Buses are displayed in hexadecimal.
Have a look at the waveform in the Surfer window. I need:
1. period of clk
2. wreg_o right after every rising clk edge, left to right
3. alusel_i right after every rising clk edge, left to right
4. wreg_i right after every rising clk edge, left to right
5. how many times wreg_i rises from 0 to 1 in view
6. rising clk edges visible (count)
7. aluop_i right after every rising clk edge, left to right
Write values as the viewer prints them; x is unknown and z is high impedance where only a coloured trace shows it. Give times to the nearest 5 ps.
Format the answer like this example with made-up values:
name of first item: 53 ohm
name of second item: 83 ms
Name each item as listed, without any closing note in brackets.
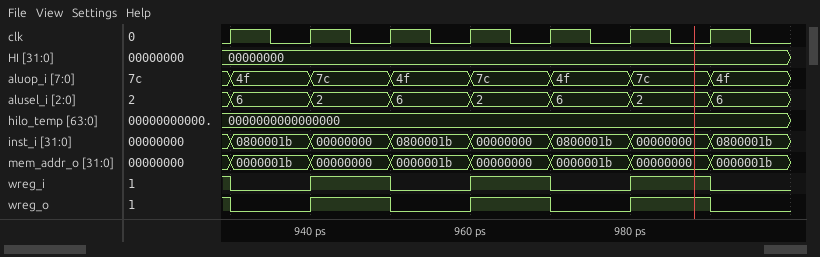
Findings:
period of clk: 10 ps
wreg_o right after every rising clk edge, left to right: 0 1 0 1 0 1 0
alusel_i right after every rising clk edge, left to right: 6, 2, 6, 2, 6, 2, 6
wreg_i right after every rising clk edge, left to right: 0 1 0 1 0 1 0
how many times wreg_i rises from 0 to 1 in view: 3
rising clk edges visible: 7
aluop_i right after every rising clk edge, left to right: 4f, 7c, 4f, 7c, 4f, 7c, 4f
